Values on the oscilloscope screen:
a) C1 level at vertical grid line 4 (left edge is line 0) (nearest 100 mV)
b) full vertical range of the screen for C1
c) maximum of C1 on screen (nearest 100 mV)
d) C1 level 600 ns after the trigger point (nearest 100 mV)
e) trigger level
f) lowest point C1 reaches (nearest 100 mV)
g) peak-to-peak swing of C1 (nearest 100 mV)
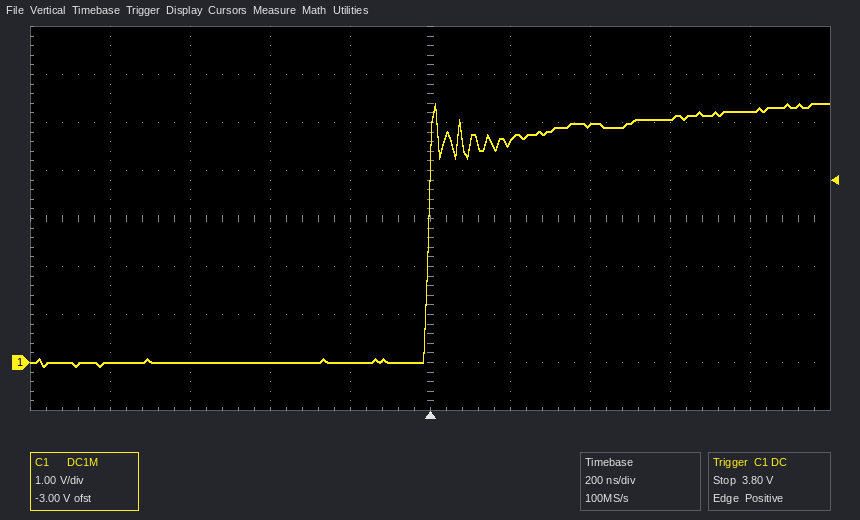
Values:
0.0 V
8 V
5.4 V
5.1 V
3.80 V
-100 mV
5.5 V
